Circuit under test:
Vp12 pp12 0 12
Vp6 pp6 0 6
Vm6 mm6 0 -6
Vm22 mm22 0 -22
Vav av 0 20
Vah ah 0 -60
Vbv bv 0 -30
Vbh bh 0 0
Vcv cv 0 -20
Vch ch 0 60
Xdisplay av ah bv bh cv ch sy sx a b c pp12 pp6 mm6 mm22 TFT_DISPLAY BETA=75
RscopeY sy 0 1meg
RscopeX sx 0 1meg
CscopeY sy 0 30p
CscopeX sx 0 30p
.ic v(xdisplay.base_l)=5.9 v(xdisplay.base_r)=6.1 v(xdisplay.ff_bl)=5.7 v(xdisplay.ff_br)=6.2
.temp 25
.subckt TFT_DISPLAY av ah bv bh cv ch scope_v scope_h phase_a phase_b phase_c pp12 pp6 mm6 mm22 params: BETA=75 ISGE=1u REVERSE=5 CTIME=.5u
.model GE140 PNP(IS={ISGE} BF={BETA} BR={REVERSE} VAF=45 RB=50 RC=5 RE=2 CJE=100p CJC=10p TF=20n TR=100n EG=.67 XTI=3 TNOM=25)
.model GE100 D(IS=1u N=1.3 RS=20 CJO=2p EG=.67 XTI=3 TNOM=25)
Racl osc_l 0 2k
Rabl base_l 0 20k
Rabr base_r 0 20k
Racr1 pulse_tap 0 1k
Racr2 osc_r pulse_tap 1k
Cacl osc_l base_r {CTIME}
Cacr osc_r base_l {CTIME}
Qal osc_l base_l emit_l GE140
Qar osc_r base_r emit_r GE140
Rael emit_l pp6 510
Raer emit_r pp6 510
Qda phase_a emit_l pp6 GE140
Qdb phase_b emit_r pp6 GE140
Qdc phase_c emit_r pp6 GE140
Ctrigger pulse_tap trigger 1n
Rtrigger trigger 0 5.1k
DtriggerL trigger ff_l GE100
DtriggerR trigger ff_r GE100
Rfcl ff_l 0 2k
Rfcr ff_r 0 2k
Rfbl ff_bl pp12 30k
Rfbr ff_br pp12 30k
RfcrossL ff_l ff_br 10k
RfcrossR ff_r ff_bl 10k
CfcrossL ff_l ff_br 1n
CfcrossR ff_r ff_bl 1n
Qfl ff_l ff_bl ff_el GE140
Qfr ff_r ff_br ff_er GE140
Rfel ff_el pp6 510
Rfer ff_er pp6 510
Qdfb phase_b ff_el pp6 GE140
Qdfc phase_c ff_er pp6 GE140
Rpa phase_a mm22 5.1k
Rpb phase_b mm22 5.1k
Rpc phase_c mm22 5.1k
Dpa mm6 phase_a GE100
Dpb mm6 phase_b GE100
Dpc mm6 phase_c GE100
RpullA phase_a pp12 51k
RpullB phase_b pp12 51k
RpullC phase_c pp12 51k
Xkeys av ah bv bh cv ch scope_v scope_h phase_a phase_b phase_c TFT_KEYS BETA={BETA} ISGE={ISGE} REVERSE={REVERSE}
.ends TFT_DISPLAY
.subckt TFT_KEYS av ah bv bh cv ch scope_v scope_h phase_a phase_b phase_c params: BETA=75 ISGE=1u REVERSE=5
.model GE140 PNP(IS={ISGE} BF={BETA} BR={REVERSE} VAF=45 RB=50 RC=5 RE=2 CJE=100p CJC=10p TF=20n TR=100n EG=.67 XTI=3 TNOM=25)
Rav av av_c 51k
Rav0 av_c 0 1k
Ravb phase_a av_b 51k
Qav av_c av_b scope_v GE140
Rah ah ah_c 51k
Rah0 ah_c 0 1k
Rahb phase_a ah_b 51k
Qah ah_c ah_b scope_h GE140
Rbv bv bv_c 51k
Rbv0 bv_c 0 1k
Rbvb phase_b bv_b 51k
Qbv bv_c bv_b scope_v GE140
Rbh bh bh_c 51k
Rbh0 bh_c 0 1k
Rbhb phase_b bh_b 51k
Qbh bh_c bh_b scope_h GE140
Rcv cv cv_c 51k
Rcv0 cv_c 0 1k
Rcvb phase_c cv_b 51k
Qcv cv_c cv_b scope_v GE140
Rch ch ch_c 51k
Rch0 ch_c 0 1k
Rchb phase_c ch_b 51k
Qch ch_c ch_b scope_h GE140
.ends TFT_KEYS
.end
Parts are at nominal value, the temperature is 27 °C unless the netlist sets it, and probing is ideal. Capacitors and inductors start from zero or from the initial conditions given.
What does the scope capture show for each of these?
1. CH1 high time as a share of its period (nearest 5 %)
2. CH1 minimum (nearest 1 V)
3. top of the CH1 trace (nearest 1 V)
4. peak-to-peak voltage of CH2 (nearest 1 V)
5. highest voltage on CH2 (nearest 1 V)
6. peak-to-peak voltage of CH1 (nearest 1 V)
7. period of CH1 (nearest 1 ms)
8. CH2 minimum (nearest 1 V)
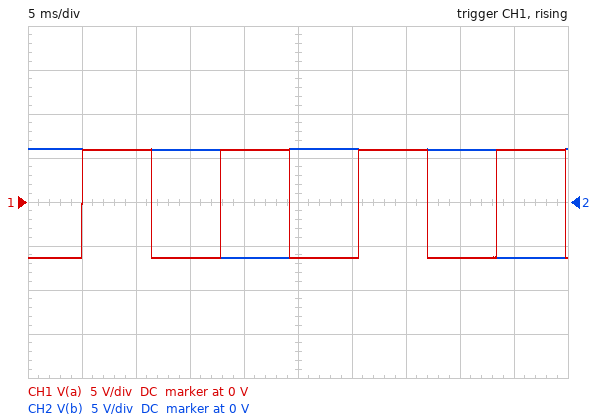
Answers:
50 %
-6 V
6 V
12 V
6 V
12 V
13 ms
-6 V
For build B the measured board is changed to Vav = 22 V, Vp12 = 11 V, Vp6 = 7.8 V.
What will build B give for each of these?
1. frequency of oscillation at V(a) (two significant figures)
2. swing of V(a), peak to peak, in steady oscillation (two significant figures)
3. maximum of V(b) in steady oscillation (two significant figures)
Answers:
77 Hz
14 V
7.8 V
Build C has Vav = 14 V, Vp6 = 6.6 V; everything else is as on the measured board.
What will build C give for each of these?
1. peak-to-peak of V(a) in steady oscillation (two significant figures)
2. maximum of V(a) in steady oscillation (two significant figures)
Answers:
13 V
6.6 V
